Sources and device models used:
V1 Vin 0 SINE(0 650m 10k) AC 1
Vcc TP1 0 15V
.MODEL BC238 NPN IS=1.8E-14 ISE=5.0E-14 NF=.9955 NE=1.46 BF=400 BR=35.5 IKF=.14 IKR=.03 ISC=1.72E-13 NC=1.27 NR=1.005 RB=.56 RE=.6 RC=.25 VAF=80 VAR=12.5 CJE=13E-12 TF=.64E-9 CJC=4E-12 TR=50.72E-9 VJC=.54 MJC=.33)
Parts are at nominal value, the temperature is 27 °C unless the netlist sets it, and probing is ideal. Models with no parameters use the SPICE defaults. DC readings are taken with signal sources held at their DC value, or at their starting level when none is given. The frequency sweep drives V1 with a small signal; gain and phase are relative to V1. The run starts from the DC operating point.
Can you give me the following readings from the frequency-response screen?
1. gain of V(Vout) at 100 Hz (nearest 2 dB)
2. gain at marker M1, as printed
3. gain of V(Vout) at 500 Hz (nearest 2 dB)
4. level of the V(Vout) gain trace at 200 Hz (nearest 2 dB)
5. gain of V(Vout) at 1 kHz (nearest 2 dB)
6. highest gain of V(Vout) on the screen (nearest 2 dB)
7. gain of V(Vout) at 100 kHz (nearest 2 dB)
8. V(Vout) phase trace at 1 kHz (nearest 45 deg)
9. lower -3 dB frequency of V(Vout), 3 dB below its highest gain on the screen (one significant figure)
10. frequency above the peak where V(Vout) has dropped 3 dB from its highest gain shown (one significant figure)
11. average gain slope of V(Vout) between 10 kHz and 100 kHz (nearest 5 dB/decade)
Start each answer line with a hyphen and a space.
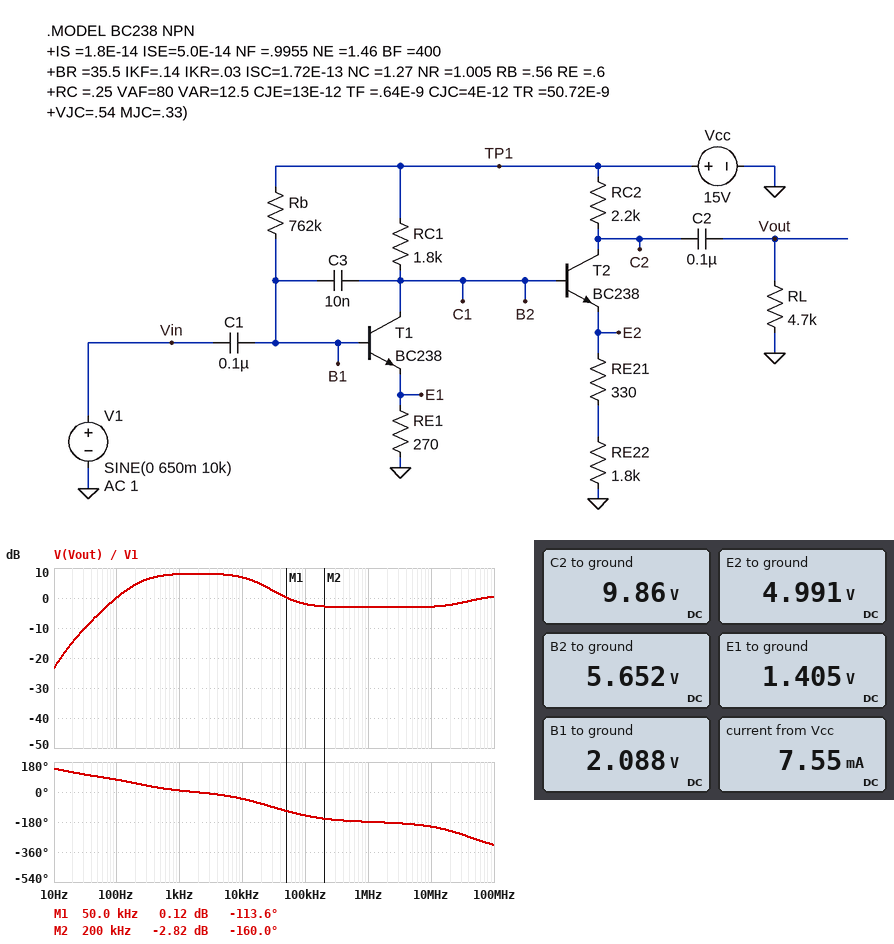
- 0 dB
- 0.12 dB
- 8 dB
- 4 dB
- 8 dB
- 8 dB
- -2 dB
- 0 deg
- 200 Hz
- 20 kHz
- -10 dB/decade
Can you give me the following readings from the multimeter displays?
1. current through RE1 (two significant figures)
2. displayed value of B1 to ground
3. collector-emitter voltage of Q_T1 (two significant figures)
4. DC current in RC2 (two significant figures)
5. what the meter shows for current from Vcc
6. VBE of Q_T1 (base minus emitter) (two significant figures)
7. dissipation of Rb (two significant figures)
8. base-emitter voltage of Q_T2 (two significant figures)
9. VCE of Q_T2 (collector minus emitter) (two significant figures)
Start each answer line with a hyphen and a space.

- 5.2 mA
- 2.088 V
- 4.2 V
- 2.3 mA
- 7.55 mA
- 680 mV
- 220 µW
- 660 mV
- 4.9 V
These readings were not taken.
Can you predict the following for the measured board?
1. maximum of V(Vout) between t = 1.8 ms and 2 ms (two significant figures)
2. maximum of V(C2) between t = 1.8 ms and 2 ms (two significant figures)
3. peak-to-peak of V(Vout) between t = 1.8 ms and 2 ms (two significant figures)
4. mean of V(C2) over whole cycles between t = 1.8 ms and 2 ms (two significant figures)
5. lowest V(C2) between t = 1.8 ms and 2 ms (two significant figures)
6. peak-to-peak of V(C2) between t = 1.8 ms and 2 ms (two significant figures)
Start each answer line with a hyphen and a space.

- 1.4 V
- 11 V
- 2.9 V
- 9.9 V
- 8.4 V
- 2.9 V
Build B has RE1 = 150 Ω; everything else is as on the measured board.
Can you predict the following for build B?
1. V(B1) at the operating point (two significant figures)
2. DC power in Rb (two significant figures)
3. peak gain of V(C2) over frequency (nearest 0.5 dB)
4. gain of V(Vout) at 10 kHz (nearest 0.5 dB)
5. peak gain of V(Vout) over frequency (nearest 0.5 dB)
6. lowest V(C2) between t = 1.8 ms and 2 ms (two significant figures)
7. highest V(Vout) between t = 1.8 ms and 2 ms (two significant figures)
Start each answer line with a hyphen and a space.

- 1.5 V
- 240 µW
- 14.0 dB
- 10.0 dB
- 11.0 dB
- 8.2 V
- 2.1 V
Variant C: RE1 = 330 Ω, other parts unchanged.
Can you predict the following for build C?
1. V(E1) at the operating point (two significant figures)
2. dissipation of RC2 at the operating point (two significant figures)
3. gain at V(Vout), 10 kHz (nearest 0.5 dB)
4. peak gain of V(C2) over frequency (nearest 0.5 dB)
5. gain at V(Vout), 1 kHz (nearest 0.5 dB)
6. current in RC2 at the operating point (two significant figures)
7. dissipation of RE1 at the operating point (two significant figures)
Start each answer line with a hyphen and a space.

- 1.7 V
- 13 mW
- 5.5 dB
- 10.0 dB
- 7.0 dB
- 2.4 mA
- 8.5 mW
